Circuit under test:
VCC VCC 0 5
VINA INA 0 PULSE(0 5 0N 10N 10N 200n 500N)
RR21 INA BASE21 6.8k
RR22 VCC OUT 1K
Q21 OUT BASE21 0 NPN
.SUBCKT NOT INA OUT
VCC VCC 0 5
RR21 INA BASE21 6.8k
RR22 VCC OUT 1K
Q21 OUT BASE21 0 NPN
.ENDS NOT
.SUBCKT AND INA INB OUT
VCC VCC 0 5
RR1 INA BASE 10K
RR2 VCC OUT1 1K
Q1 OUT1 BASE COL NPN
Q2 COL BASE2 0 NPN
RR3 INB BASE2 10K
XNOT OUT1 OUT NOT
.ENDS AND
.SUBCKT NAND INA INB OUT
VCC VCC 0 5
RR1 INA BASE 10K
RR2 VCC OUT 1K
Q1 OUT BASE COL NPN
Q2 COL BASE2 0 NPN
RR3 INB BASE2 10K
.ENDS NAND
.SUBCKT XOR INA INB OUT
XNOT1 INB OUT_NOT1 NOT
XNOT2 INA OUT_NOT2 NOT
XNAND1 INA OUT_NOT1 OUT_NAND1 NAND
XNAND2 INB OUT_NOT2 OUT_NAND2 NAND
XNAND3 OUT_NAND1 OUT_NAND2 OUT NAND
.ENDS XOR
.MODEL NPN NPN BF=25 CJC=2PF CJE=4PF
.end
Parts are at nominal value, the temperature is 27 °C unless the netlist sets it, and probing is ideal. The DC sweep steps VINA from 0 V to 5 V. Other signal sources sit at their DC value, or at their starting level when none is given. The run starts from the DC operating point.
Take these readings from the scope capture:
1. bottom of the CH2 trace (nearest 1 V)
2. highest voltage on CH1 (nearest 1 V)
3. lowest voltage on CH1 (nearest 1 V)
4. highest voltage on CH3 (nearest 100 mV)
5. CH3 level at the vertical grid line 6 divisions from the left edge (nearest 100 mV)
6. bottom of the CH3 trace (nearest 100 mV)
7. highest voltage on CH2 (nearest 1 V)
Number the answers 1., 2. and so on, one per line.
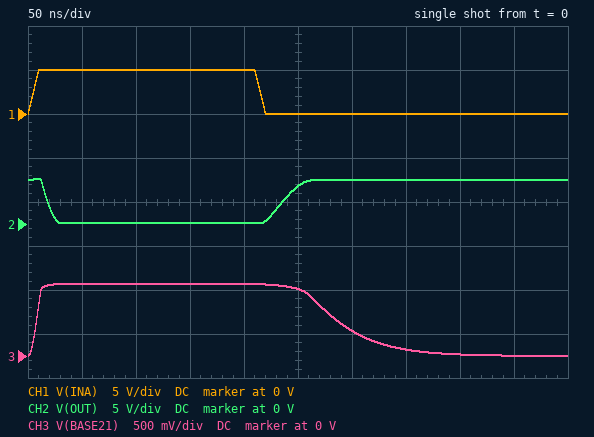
1. 0 V
2. 5 V
3. 0 V
4. 800 mV
5. 300 mV
6. 0 V
7. 5 V
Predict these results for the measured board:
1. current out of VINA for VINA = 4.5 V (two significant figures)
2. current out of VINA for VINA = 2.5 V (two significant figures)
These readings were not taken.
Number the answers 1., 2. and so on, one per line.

1. 540 µA
2. 250 µA
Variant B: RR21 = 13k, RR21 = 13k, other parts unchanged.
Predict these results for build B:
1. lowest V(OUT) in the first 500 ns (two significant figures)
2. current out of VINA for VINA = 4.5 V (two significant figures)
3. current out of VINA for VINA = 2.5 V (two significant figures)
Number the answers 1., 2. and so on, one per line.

1. 98 mV
2. 280 µA
3. 130 µA
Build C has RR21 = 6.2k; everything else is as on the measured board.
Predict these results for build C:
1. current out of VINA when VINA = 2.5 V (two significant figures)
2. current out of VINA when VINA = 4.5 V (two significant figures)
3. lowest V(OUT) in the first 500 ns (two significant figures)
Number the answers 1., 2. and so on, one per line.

1. 270 µA
2. 590 µA
3. 67 mV
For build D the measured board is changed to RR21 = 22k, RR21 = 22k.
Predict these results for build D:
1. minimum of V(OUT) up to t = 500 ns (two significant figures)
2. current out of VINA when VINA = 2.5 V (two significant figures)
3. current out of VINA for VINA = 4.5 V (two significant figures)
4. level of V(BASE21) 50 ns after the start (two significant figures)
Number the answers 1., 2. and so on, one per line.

1. 370 mV
2. 78 µA
3. 170 µA
4. 800 mV
